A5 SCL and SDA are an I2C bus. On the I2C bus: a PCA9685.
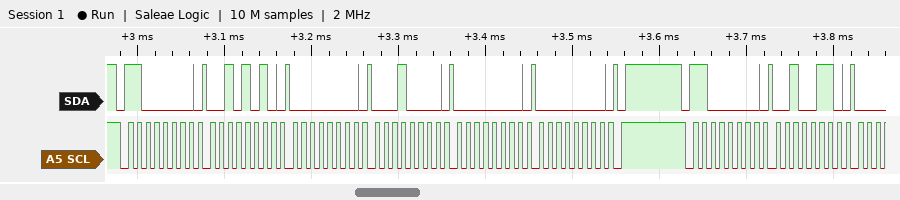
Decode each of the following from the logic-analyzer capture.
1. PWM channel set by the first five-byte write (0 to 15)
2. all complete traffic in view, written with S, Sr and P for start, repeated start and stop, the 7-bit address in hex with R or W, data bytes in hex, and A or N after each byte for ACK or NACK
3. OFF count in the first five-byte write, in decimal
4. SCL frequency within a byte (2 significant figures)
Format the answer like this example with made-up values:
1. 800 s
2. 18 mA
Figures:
1. 9
2. S 60W A 2A A 00 A 10 A 00 A 00 A P S 60W A 26 A
3. 0
4. 100 kHz
